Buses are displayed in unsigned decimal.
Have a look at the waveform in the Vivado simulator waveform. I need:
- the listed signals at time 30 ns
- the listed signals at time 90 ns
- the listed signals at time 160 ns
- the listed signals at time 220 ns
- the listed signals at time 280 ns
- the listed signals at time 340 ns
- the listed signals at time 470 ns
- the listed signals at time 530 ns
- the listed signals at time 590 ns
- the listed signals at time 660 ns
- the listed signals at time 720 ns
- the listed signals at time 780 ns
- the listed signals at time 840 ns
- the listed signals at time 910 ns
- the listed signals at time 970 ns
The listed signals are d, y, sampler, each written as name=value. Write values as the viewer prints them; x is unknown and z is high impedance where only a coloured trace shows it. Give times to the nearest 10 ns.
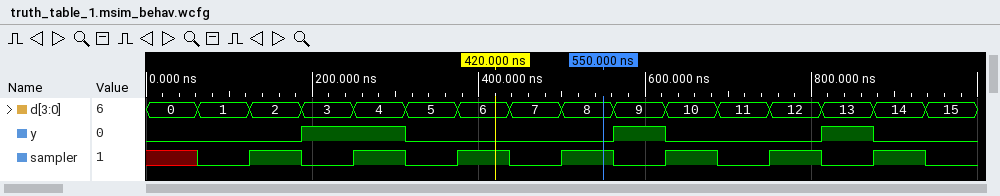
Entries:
d=0, y=0, sampler=x
d=1, y=0, sampler=0
d=2, y=0, sampler=1
d=3, y=1, sampler=0
d=4, y=1, sampler=1
d=5, y=0, sampler=0
d=7, y=0, sampler=0
d=8, y=0, sampler=1
d=9, y=1, sampler=0
d=10, y=0, sampler=1
d=11, y=0, sampler=0
d=12, y=0, sampler=1
d=13, y=1, sampler=0
d=14, y=0, sampler=1
d=15, y=0, sampler=0
